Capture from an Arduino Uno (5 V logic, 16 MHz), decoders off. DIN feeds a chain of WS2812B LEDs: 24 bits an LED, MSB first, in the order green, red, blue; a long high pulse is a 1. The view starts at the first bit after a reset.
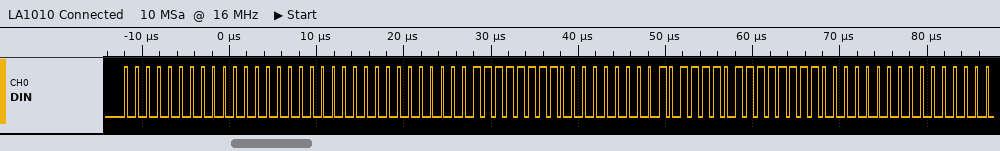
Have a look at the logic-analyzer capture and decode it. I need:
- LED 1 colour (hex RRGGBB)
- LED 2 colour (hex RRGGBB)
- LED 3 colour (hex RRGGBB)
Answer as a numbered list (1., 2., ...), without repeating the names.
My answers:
1. #000000
2. #FF0000
3. #FF5E00
